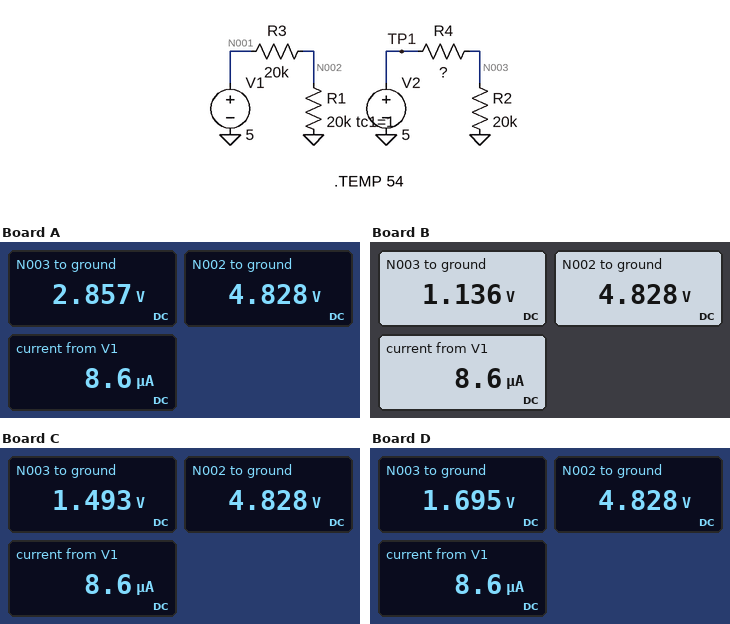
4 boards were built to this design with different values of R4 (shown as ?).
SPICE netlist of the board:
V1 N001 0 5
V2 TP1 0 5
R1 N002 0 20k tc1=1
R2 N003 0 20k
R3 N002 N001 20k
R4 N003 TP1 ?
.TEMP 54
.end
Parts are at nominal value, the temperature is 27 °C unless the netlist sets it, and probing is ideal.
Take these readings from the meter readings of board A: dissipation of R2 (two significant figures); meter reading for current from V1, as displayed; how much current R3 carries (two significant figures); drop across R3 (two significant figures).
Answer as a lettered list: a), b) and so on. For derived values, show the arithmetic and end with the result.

a) (2.857 V)^2 / 20 kΩ = 410 µW
b) 8.6 µA
c) (5 V - 4.828 V) / 20 kΩ = 8.6 µA
d) 5 V - 4.828 V = 170 mV
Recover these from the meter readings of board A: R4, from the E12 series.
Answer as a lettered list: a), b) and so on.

a) 15 kΩ
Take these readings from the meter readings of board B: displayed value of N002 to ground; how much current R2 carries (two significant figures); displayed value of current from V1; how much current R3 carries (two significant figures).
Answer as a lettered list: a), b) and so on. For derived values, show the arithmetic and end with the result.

a) 4.828 V
b) (1.136 V) / 20 kΩ = 57 µA
c) 8.6 µA
d) (5 V - 4.828 V) / 20 kΩ = 8.6 µA
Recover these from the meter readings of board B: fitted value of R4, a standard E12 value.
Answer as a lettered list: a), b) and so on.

a) 68 kΩ
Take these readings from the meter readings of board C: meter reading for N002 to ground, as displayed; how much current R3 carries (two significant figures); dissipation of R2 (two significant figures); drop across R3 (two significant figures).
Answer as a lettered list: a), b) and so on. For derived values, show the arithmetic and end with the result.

a) 4.828 V
b) (5 V - 4.828 V) / 20 kΩ = 8.6 µA
c) (1.493 V)^2 / 20 kΩ = 110 µW
d) 5 V - 4.828 V = 170 mV
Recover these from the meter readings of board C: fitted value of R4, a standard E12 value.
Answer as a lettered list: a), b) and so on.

a) 47 kΩ
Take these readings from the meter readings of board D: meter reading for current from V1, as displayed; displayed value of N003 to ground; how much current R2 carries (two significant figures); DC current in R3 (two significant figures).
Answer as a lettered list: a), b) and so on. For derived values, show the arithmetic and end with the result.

a) 8.6 µA
b) 1.695 V
c) (1.695 V) / 20 kΩ = 85 µA
d) (5 V - 4.828 V) / 20 kΩ = 8.6 µA
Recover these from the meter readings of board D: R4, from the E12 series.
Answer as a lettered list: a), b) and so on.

a) 39 kΩ
